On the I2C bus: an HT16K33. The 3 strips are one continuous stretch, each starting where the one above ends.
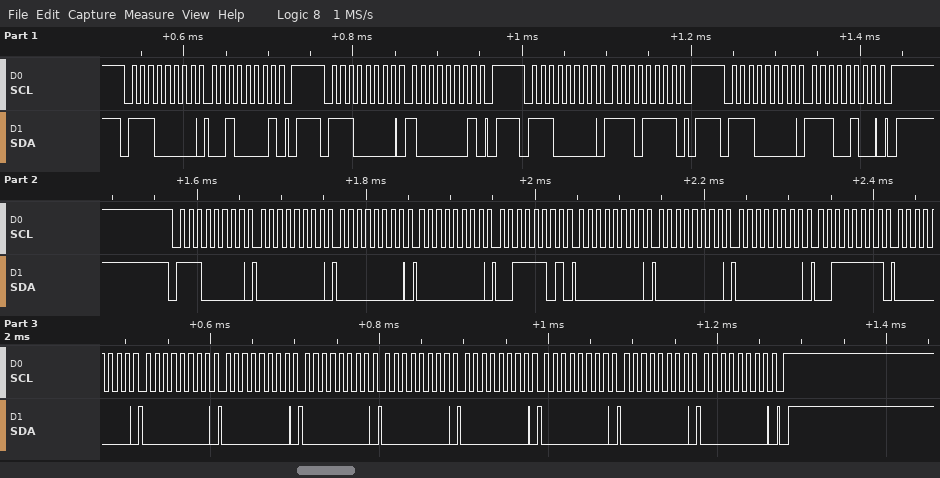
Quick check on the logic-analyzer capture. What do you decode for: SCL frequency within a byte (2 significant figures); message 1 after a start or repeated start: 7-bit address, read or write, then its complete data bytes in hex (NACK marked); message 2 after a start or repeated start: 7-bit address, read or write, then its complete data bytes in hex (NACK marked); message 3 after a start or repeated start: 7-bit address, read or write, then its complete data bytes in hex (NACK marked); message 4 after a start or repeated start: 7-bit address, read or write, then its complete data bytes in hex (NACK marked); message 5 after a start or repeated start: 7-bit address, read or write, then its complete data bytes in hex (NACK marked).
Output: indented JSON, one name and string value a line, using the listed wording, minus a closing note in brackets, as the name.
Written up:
{
  "SCL frequency within a byte": "100 kHz",
  "message 1 after a start or repeated start: 7-bit address, read or write, then its complete data bytes in hex": "0x70 write: 21",
  "message 2 after a start or repeated start: 7-bit address, read or write, then its complete data bytes in hex": "0x70 write: 81",
  "message 3 after a start or repeated start: 7-bit address, read or write, then its complete data bytes in hex": "0x70 write: EF",
  "message 4 after a start or repeated start: 7-bit address, read or write, then its complete data bytes in hex": "0x70 write: E4",
  "message 5 after a start or repeated start: 7-bit address, read or write, then its complete data bytes in hex": "0x70 write: 00 00 00 3D 00 00 00 3F 00 00 00 00 00 00 00 00 00"
}
